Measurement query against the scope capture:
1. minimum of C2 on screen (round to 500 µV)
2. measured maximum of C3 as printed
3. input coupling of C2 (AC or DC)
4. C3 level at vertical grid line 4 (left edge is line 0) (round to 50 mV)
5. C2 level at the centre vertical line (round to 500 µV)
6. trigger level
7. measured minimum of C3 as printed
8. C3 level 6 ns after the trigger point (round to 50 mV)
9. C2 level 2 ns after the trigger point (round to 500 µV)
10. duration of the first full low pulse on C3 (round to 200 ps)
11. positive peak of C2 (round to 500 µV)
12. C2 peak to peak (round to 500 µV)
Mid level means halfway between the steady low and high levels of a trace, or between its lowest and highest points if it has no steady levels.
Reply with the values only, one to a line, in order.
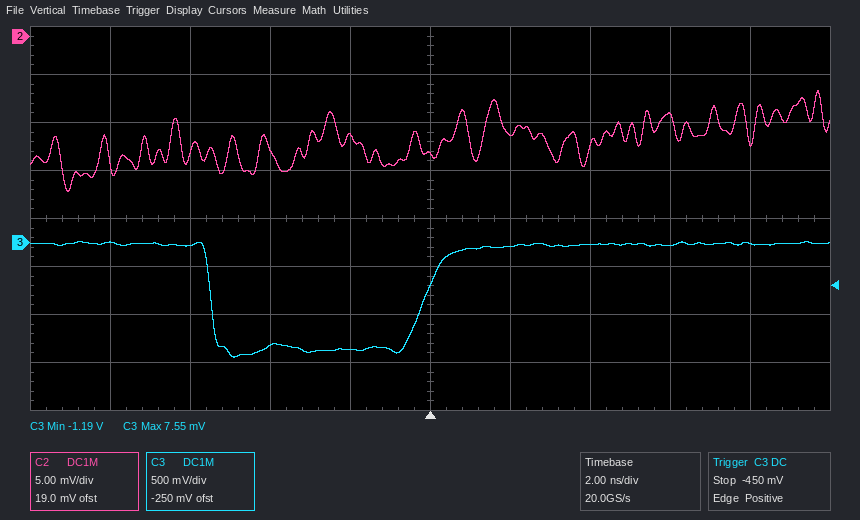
-16.0 mV
7.55 mV
DC
-1.10 V
-12.5 mV
-450 mV
-1.19 V
-50 mV
-10.0 mV
5.4 ns
-5.5 mV
10.5 mV
